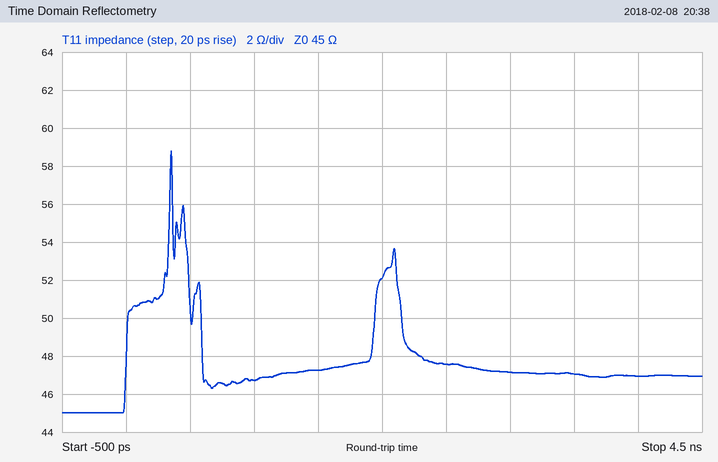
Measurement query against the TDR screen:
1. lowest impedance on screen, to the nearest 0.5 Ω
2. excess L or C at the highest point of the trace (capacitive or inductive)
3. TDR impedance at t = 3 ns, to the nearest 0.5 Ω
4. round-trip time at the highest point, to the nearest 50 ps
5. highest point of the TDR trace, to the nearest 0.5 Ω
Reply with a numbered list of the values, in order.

1. 45.0 Ω
2. inductive
3. 47.0 Ω
4. 350 ps
5. 59.0 Ω
